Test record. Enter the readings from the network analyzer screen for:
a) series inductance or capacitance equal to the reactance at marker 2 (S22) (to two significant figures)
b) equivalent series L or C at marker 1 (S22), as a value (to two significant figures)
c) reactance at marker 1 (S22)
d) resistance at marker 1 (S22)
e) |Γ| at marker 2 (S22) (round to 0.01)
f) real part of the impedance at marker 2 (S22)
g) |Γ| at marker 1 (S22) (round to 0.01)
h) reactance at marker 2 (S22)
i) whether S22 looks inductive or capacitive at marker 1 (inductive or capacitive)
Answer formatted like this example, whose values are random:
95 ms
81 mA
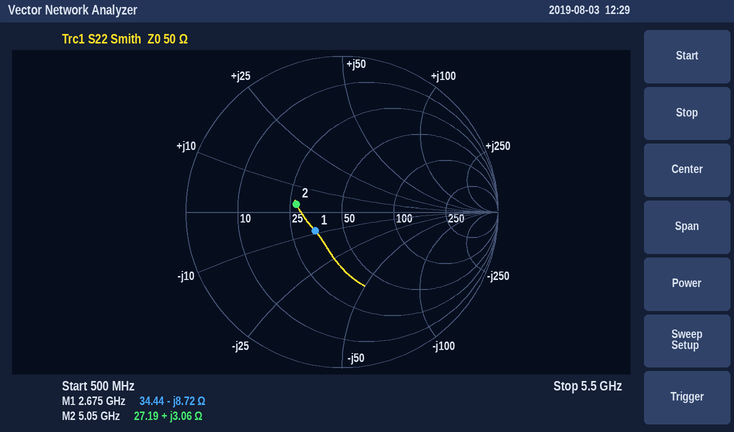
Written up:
96 pH
6.8 pF
-8.72 Ω
34.44 Ω
0.30
27.19 Ω
0.21
+3.06 Ω
capacitive
